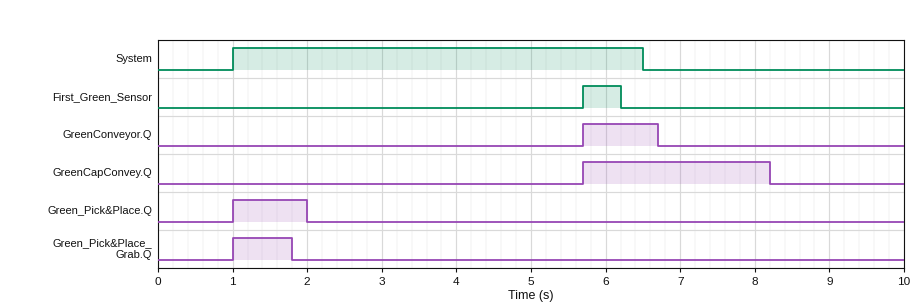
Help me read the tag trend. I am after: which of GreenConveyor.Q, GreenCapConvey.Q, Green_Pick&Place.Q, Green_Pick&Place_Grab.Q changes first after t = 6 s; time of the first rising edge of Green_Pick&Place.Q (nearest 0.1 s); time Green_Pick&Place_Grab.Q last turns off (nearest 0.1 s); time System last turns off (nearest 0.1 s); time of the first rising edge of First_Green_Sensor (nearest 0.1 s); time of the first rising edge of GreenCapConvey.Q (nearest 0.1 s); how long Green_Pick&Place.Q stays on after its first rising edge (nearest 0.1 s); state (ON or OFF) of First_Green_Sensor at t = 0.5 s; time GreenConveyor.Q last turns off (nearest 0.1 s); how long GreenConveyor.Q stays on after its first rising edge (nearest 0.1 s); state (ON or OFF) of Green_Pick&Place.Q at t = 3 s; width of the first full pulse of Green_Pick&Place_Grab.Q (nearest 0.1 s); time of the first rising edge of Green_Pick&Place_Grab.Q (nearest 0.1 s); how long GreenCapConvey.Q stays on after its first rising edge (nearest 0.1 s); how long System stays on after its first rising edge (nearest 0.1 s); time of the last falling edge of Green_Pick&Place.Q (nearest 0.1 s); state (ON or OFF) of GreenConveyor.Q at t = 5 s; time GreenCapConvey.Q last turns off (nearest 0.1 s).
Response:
GreenConveyor.Q
1.0 s
1.8 s
6.5 s
5.7 s
5.7 s
1.0 s
OFF
6.7 s
1.0 s
OFF
0.8 s
1.0 s
2.5 s
5.5 s
2.0 s
OFF
8.2 s
